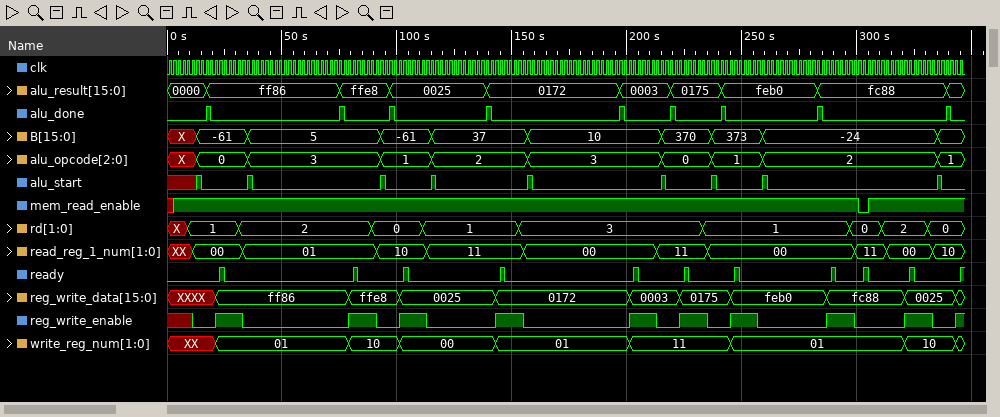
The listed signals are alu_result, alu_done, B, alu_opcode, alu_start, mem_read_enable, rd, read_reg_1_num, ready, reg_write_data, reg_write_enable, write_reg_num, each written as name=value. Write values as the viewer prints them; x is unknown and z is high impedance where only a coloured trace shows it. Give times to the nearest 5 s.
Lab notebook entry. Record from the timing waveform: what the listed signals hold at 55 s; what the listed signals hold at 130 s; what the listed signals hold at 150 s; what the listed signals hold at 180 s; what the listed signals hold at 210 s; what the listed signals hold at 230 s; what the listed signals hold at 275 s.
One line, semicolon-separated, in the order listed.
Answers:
alu_result=ff86, alu_done=0, B=5, alu_opcode=3, alu_start=0, mem_read_enable=1, rd=2, read_reg_1_num=01, ready=0, reg_write_data=ff86, reg_write_enable=0, write_reg_num=01; alu_result=0025, alu_done=0, B=37, alu_opcode=2, alu_start=0, mem_read_enable=1, rd=1, read_reg_1_num=11, ready=0, reg_write_data=0025, reg_write_enable=0, write_reg_num=00; alu_result=0172, alu_done=0, B=37, alu_opcode=2, alu_start=0, mem_read_enable=1, rd=1, read_reg_1_num=11, ready=0, reg_write_data=0172, reg_write_enable=1, write_reg_num=01; alu_result=0172, alu_done=0, B=10, alu_opcode=3, alu_start=0, mem_read_enable=1, rd=3, read_reg_1_num=00, ready=0, reg_write_data=0172, reg_write_enable=0, write_reg_num=01; alu_result=0003, alu_done=0, B=10, alu_opcode=3, alu_start=0, mem_read_enable=1, rd=3, read_reg_1_num=00, ready=0, reg_write_data=0003, reg_write_enable=1, write_reg_num=11; alu_result=0175, alu_done=0, B=370, alu_opcode=0, alu_start=0, mem_read_enable=1, rd=3, read_reg_1_num=11, ready=0, reg_write_data=0175, reg_write_enable=1, write_reg_num=11; alu_result=feb0, alu_done=0, B=-24, alu_opcode=2, alu_start=0, mem_read_enable=1, rd=1, read_reg_1_num=00, ready=0, reg_write_data=feb0, reg_write_enable=0, write_reg_num=01
